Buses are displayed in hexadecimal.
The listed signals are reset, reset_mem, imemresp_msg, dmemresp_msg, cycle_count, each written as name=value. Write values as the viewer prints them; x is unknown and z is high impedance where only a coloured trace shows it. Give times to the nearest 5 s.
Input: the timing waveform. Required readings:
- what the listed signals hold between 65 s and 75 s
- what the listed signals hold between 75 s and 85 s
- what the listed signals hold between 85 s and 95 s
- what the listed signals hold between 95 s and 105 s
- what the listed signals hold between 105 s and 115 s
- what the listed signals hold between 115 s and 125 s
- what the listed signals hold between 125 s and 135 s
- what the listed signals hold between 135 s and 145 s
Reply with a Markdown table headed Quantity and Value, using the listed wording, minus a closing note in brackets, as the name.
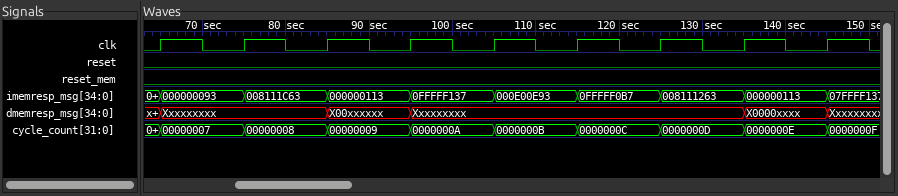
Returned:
| Quantity | Value |
|---|---|
| what the listed signals hold between 65 s and 75 s | reset=0, reset_mem=0, imemresp_msg=000000093, dmemresp_msg=Xxxxxxxxx, cycle_count=00000007 |
| what the listed signals hold between 75 s and 85 s | reset=0, reset_mem=0, imemresp_msg=008111C63, dmemresp_msg=Xxxxxxxxx, cycle_count=00000008 |
| what the listed signals hold between 85 s and 95 s | reset=0, reset_mem=0, imemresp_msg=000000113, dmemresp_msg=X00xxxxxx, cycle_count=00000009 |
| what the listed signals hold between 95 s and 105 s | reset=0, reset_mem=0, imemresp_msg=0FFFFF137, dmemresp_msg=Xxxxxxxxx, cycle_count=0000000A |
| what the listed signals hold between 105 s and 115 s | reset=0, reset_mem=0, imemresp_msg=000E00E93, dmemresp_msg=Xxxxxxxxx, cycle_count=0000000B |
| what the listed signals hold between 115 s and 125 s | reset=0, reset_mem=0, imemresp_msg=0FFFFF0B7, dmemresp_msg=Xxxxxxxxx, cycle_count=0000000C |
| what the listed signals hold between 125 s and 135 s | reset=0, reset_mem=0, imemresp_msg=008111263, dmemresp_msg=Xxxxxxxxx, cycle_count=0000000D |
| what the listed signals hold between 135 s and 145 s | reset=0, reset_mem=0, imemresp_msg=000000113, dmemresp_msg=X0000xxxx, cycle_count=0000000E |
